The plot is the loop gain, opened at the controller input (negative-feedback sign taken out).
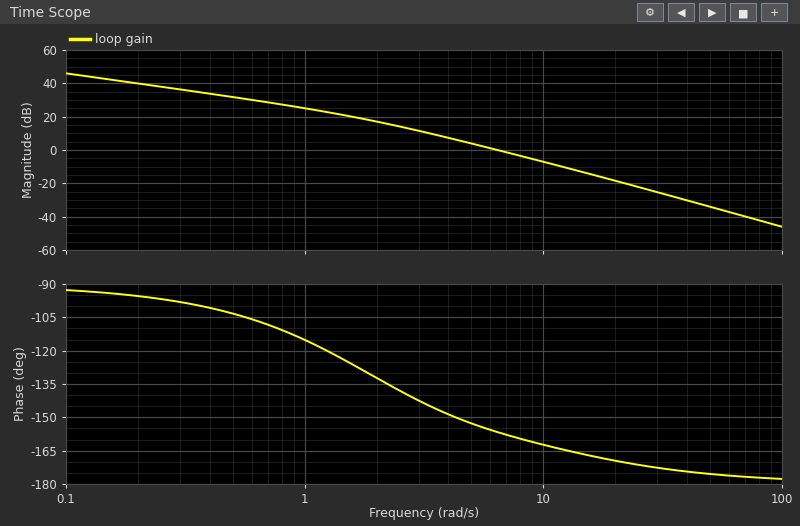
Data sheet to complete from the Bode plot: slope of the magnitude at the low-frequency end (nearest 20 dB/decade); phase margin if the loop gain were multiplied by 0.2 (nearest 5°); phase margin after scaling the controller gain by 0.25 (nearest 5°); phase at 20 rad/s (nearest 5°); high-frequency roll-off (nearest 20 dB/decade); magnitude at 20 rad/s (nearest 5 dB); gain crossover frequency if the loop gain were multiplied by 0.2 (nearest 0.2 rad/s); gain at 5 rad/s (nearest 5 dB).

-20 dB/decade
40°
40°
-170°
-40 dB/decade
-20 dB
2.6 rad/s
5 dB
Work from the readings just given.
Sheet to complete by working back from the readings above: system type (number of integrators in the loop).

1
